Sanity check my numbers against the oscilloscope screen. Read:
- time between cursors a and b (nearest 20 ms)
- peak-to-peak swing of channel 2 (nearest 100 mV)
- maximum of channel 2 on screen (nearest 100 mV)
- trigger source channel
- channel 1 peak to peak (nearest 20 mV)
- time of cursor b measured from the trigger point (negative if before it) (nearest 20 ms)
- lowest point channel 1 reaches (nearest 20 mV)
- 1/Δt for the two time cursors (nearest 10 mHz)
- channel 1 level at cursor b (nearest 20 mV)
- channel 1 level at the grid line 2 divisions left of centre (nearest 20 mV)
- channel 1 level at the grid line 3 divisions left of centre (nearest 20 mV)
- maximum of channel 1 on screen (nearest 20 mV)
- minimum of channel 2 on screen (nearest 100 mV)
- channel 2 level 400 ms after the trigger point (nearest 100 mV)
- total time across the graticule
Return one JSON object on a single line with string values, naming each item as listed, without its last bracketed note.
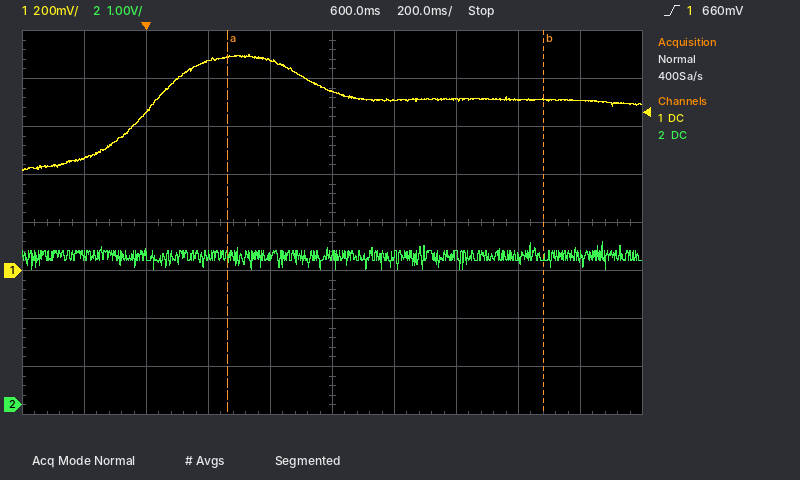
{"time between cursors a and b": "1.02 s", "peak-to-peak swing of channel 2": "600 mV", "maximum of channel 2 on screen": "3.4 V", "trigger source channel": "channel 1", "channel 1 peak to peak": "480 mV", "time of cursor b measured from the trigger point (negative if before it)": "+1.28 s", "lowest point channel 1 reaches": "420 mV", "1/Δt for the two time cursors": "980 mHz", "channel 1 level at cursor b": "720 mV", "channel 1 level at the grid line 2 divisions left of centre": "880 mV", "channel 1 level at the grid line 3 divisions left of centre": "660 mV", "maximum of channel 1 on screen": "900 mV", "minimum of channel 2 on screen": "2.8 V", "channel 2 level 400 ms after the trigger point": "3.1 V", "total time across the graticule": "2 s"}
